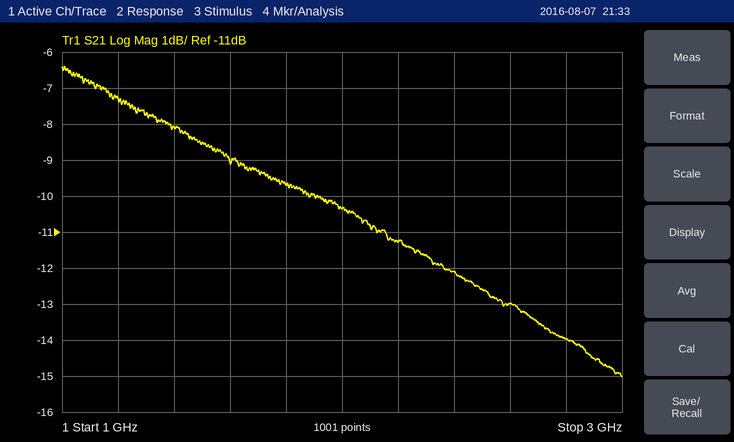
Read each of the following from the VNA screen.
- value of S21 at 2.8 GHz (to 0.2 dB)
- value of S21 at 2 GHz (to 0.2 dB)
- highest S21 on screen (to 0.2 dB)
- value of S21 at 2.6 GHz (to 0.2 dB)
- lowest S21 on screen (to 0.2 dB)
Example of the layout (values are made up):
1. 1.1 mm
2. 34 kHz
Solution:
1. -14.0 dB
2. -10.4 dB
3. -6.4 dB
4. -13.0 dB
5. -15.0 dB
